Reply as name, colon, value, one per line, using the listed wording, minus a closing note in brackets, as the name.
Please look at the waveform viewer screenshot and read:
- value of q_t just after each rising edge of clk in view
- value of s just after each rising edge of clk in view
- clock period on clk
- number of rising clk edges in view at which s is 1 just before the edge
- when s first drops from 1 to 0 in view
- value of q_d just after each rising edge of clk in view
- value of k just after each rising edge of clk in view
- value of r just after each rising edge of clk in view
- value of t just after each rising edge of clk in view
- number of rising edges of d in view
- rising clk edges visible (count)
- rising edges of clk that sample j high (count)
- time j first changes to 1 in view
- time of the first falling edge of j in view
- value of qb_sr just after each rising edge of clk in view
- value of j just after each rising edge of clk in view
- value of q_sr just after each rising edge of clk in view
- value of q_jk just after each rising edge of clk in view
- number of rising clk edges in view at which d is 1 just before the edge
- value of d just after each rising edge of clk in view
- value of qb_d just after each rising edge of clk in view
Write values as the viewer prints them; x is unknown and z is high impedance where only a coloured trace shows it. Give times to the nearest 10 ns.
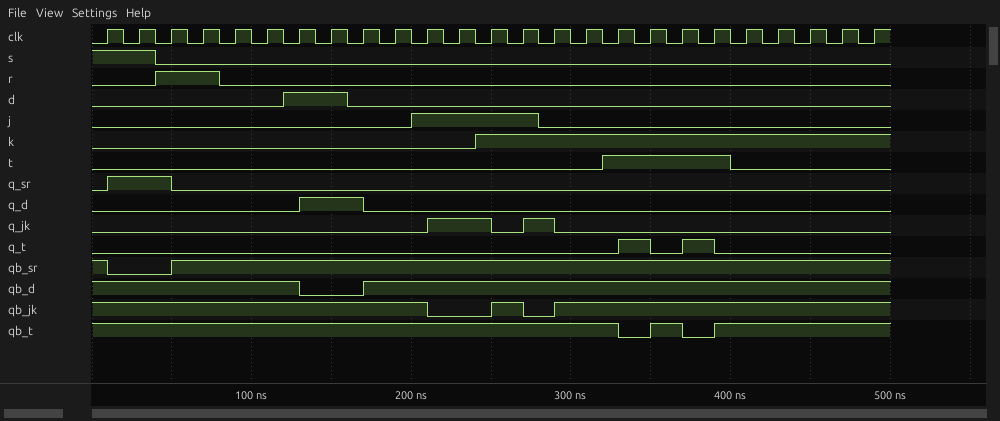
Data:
value of q_t just after each rising edge of clk in view: 0 0 0 0 0 0 0 0 0 0 0 0 0 0 0 0 1 0 1 0 0 0 0 0 0
value of s just after each rising edge of clk in view: 1 1 0 0 0 0 0 0 0 0 0 0 0 0 0 0 0 0 0 0 0 0 0 0 0
clock period on clk: 20 ns
number of rising clk edges in view at which s is 1 just before the edge: 2
when s first drops from 1 to 0 in view: 40 ns
value of q_d just after each rising edge of clk in view: 0 0 0 0 0 0 1 1 0 0 0 0 0 0 0 0 0 0 0 0 0 0 0 0 0
value of k just after each rising edge of clk in view: 0 0 0 0 0 0 0 0 0 0 0 0 1 1 1 1 1 1 1 1 1 1 1 1 1
value of r just after each rising edge of clk in view: 0 0 1 1 0 0 0 0 0 0 0 0 0 0 0 0 0 0 0 0 0 0 0 0 0
value of t just after each rising edge of clk in view: 0 0 0 0 0 0 0 0 0 0 0 0 0 0 0 0 1 1 1 1 0 0 0 0 0
number of rising edges of d in view: 1
rising clk edges visible: 25
rising edges of clk that sample j high: 4
time j first changes to 1 in view: 200 ns
time of the first falling edge of j in view: 280 ns
value of qb_sr just after each rising edge of clk in view: 0 0 1 1 1 1 1 1 1 1 1 1 1 1 1 1 1 1 1 1 1 1 1 1 1
value of j just after each rising edge of clk in view: 0 0 0 0 0 0 0 0 0 0 1 1 1 1 0 0 0 0 0 0 0 0 0 0 0
value of q_sr just after each rising edge of clk in view: 1 1 0 0 0 0 0 0 0 0 0 0 0 0 0 0 0 0 0 0 0 0 0 0 0
value of q_jk just after each rising edge of clk in view: 0 0 0 0 0 0 0 0 0 0 1 1 0 1 0 0 0 0 0 0 0 0 0 0 0
number of rising clk edges in view at which d is 1 just before the edge: 2
value of d just after each rising edge of clk in view: 0 0 0 0 0 0 1 1 0 0 0 0 0 0 0 0 0 0 0 0 0 0 0 0 0
value of qb_d just after each rising edge of clk in view: 1 1 1 1 1 1 0 0 1 1 1 1 1 1 1 1 1 1 1 1 1 1 1 1 1
